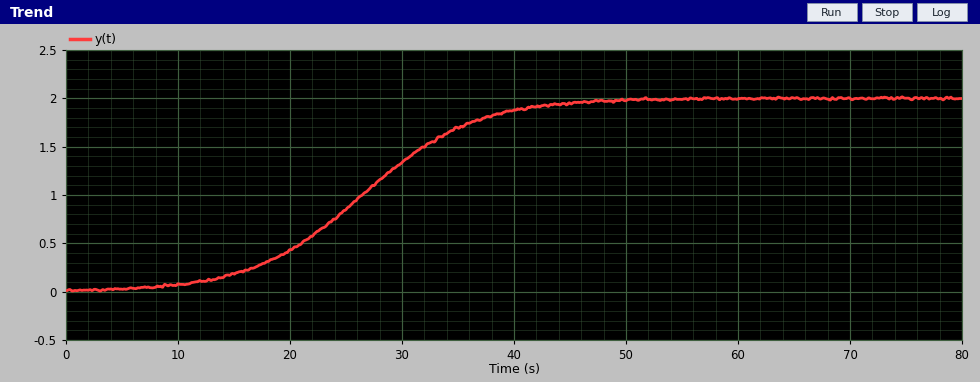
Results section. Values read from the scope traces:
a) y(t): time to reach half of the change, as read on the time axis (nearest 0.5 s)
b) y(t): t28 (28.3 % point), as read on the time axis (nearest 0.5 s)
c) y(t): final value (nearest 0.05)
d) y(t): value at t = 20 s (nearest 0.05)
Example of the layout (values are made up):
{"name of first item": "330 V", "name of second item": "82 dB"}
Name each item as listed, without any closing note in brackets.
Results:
{"y(t): time to reach half of the change, as read on the time axis": "26.5 s", "y(t): t28 (28.3 % point), as read on the time axis": "22.0 s", "y(t): final value": "2.00", "y(t): value at t = 20 s": "0.45"}
